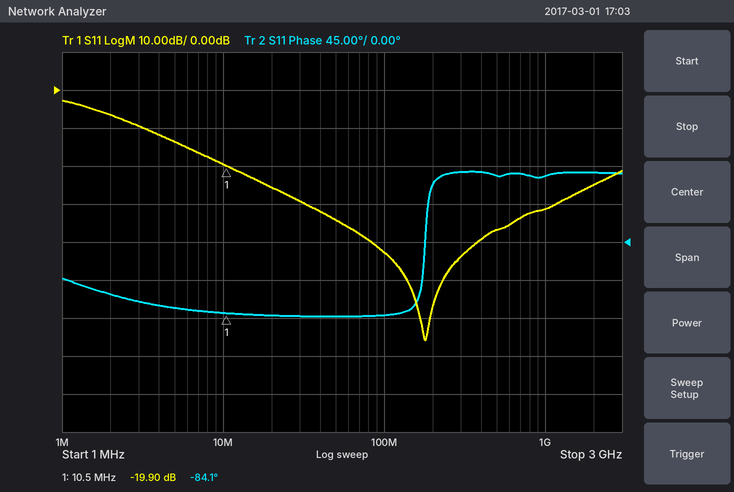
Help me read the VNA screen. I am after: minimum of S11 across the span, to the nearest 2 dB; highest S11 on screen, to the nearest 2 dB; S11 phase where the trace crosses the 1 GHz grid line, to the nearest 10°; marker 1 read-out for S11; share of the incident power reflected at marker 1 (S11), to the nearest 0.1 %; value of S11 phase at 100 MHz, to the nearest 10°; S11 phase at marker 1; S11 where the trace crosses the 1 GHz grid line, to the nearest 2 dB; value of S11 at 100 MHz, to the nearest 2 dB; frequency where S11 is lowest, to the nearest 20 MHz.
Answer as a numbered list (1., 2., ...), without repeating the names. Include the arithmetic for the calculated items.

1. -66 dB
2. -2 dB
3. 80°
4. -19.90 dB
5. 10^(-19.9/10) ≈ 1.0 %
6. -90°
7. -84.1°
8. -32 dB
9. -42 dB
10. 180 MHz
